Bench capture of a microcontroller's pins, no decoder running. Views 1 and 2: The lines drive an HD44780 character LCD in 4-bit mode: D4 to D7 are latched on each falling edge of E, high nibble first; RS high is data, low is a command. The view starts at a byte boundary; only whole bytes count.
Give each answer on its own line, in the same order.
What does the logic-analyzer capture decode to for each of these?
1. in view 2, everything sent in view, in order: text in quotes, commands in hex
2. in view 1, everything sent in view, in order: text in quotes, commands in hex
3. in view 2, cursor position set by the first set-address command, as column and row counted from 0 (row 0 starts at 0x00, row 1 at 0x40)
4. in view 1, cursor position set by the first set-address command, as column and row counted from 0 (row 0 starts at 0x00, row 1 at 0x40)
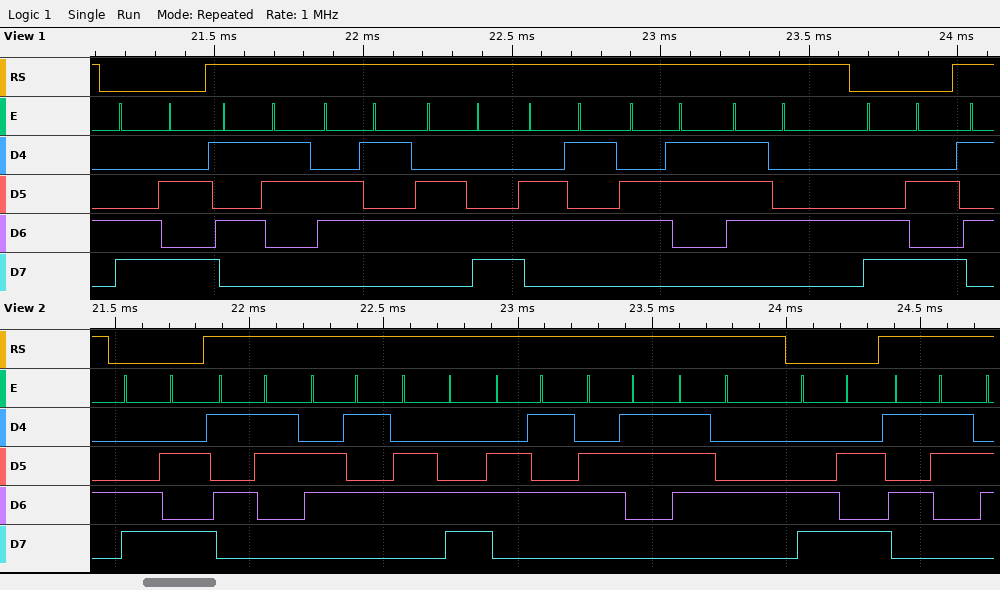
0xCA "Select" 0xCA "S"
0xCA "Select" 0xCA
column 10, row 1
column 10, row 1
